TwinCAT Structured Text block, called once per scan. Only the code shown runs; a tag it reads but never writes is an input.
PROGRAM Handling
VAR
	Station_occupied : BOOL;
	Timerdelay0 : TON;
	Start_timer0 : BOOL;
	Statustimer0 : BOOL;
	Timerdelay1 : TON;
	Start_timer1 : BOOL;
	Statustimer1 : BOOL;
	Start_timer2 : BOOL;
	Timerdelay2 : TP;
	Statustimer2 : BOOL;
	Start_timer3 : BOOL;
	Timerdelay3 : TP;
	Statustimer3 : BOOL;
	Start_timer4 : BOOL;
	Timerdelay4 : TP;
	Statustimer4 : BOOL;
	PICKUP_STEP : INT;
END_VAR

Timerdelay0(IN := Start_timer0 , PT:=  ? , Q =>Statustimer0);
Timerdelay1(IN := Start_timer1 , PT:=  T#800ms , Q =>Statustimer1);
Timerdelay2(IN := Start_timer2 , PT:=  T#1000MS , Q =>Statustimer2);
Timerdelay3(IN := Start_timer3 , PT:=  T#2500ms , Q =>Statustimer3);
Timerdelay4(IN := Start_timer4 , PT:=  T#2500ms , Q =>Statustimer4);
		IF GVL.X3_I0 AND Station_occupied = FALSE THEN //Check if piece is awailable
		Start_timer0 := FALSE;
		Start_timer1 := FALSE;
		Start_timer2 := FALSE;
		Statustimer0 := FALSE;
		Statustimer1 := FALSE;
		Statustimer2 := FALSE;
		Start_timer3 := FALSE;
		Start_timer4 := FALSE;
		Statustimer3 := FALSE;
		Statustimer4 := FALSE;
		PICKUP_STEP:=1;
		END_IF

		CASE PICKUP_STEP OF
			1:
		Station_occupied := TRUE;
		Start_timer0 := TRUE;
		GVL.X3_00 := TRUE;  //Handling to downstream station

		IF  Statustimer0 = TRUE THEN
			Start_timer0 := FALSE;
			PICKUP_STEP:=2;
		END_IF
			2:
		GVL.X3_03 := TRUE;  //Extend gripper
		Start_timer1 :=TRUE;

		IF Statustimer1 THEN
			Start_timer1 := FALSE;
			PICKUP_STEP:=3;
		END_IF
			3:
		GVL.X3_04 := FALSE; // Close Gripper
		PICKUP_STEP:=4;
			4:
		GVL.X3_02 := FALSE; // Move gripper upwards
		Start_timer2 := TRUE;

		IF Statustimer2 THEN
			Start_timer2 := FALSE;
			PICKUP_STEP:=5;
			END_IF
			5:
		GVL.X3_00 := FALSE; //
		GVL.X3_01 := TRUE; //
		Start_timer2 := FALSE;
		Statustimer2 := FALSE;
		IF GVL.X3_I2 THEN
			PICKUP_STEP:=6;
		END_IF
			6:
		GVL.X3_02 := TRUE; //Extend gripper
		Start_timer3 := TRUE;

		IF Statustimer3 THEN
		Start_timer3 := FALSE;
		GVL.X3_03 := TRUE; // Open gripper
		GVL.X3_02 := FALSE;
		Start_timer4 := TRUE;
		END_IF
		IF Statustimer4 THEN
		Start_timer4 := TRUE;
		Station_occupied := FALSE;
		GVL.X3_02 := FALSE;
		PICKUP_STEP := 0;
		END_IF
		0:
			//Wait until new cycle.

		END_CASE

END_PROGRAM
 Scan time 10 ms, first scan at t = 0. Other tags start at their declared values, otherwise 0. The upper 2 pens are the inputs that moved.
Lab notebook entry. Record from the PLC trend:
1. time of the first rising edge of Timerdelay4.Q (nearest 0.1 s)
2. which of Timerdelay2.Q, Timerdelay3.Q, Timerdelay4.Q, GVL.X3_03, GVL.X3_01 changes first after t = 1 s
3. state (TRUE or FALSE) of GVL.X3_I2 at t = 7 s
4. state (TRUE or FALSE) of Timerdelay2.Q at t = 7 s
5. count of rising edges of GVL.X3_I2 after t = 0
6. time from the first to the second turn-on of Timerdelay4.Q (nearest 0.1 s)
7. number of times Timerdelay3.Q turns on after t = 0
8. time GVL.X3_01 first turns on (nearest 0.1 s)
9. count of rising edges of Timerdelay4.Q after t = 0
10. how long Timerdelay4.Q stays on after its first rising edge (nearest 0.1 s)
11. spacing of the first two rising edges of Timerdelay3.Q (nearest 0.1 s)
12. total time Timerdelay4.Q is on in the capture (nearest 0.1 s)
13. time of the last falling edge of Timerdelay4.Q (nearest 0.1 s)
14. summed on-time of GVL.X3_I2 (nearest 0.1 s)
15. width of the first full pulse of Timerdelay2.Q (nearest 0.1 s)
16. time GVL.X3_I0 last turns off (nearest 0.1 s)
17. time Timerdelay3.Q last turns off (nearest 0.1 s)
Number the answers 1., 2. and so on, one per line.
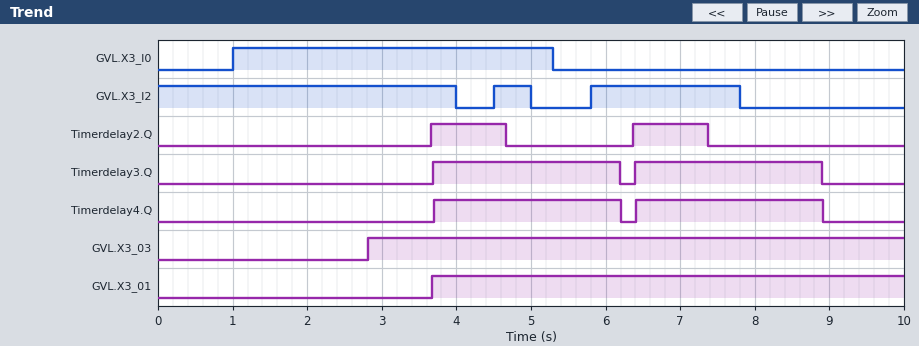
1. 3.7 s
2. GVL.X3_03
3. TRUE
4. TRUE
5. 2
6. 2.7 s
7. 2
8. 3.7 s
9. 2
10. 2.5 s
11. 2.7 s
12. 5.0 s
13. 8.9 s
14. 6.5 s
15. 1.0 s
16. 5.3 s
17. 8.9 s
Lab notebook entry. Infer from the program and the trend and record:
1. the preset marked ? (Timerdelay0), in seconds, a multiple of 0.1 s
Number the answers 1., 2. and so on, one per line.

1. 1.8 s
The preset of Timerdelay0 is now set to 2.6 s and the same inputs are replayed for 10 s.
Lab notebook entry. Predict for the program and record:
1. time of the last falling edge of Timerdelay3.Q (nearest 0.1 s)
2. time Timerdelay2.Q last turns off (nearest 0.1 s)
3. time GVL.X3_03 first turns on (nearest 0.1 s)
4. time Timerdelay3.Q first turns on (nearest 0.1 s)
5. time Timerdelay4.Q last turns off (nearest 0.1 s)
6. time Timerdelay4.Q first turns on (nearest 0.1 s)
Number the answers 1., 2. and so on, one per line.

1. 7.0 s
2. 9.0 s
3. 3.6 s
4. 4.5 s
5. 7.0 s
6. 4.5 s
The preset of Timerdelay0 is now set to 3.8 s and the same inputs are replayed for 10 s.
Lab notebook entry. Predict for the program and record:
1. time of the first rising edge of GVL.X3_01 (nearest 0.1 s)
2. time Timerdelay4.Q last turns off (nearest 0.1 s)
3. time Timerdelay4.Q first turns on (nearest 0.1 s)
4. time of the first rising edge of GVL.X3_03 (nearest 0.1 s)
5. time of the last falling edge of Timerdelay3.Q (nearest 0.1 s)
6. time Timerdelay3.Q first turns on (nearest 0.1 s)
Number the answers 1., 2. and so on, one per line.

1. 5.7 s
2. 8.3 s
3. 5.8 s
4. 4.8 s
5. 8.3 s
6. 5.8 s
